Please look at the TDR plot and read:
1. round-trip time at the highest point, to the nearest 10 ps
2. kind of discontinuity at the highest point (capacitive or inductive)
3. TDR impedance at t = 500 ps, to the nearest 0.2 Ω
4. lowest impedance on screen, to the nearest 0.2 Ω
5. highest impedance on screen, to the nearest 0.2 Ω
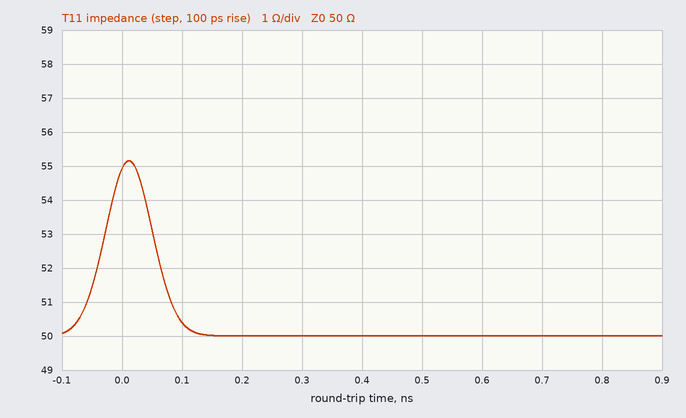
10 ps
inductive
50.0 Ω
50.0 Ω
55.2 Ω
